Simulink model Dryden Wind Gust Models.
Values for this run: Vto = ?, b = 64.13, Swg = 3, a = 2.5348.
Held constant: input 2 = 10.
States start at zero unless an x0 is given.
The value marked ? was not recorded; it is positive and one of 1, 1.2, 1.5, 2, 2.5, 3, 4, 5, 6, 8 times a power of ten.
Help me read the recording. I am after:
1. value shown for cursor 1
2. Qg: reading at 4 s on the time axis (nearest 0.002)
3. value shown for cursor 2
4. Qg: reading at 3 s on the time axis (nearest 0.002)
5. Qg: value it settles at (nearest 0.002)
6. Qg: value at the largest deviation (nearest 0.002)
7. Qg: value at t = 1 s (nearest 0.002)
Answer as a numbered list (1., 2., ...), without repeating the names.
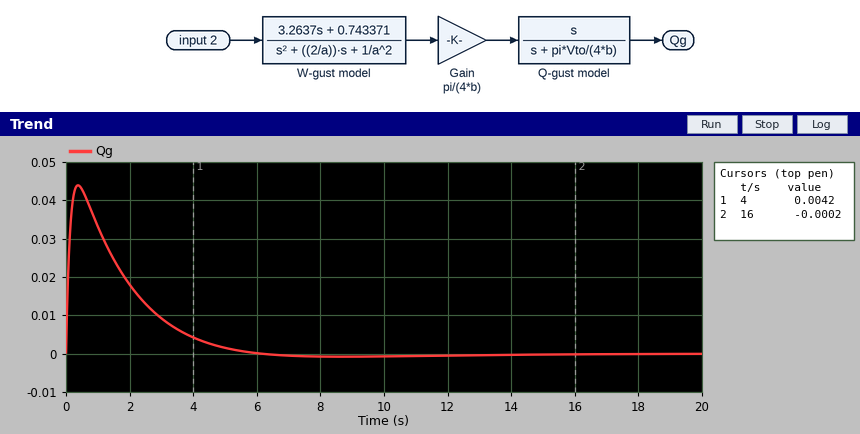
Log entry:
1. 0.0042
2. 0.004
3. -0.0002
4. 0.010
5. 0.000
6. 0.044
7. 0.034
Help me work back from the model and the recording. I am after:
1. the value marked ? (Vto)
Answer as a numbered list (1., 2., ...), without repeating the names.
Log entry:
1. 600
